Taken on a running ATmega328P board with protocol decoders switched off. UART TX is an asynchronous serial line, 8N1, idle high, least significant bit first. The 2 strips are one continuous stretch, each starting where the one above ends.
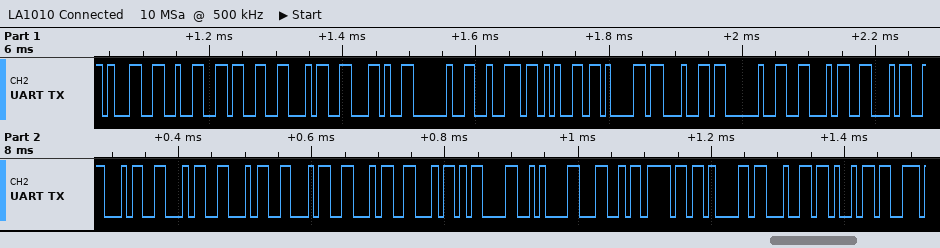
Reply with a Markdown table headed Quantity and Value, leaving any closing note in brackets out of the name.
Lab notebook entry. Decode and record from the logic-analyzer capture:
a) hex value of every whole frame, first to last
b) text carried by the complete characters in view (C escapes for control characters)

| Quantity | Value |
|---|---|
| hex value of every whole frame, first to last | 31 32 33 34 2C 20 72 65 61 64 20 46 46 46 46 46 46 46 46 0D 0A 4C 6F 61 64 69 |
| text carried by the complete characters in view | "1234, read FFFFFFFF\r\nLoadi" |
